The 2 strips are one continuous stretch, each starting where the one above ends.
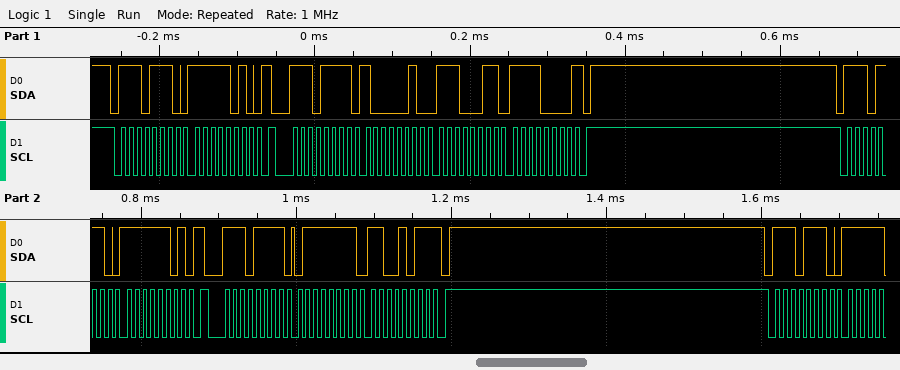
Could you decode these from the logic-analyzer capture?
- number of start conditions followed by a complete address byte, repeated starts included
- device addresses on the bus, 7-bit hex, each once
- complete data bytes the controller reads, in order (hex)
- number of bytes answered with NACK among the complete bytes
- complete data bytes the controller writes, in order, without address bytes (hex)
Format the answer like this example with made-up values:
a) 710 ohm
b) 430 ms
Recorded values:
a) 5
b) 0x77
c) 82 E3 F0 7F CB
d) 2
e) FA FD
